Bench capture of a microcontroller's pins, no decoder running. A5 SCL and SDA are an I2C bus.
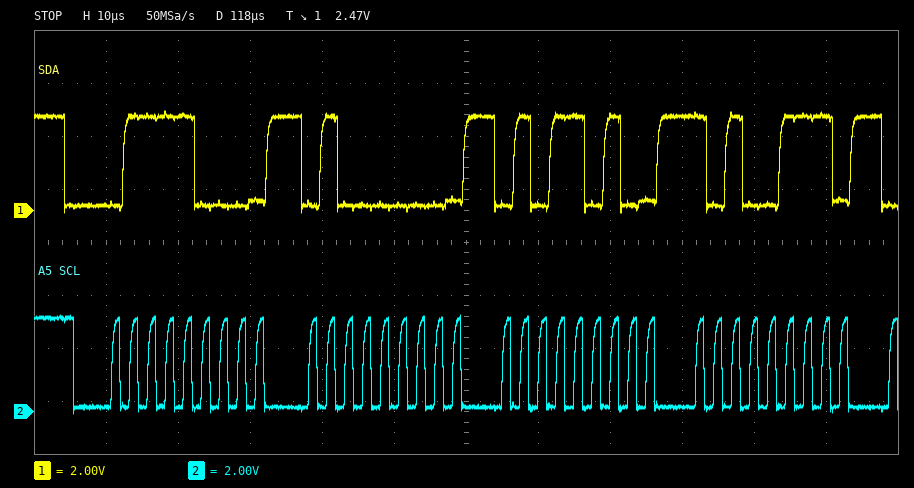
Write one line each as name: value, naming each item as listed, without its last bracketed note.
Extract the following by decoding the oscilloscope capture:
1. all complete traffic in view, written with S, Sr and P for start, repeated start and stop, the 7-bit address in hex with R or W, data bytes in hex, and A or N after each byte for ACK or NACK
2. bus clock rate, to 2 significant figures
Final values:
all complete traffic in view, written with S, Sr and P for start, repeated start and stop, the 7-bit address in hex with R or W, data bytes in hex, and A or N after each byte for ACK or NACK: S 3CW A 40 A 5A A A7 A
bus clock rate, to 2 significant figures: 400 kHz
